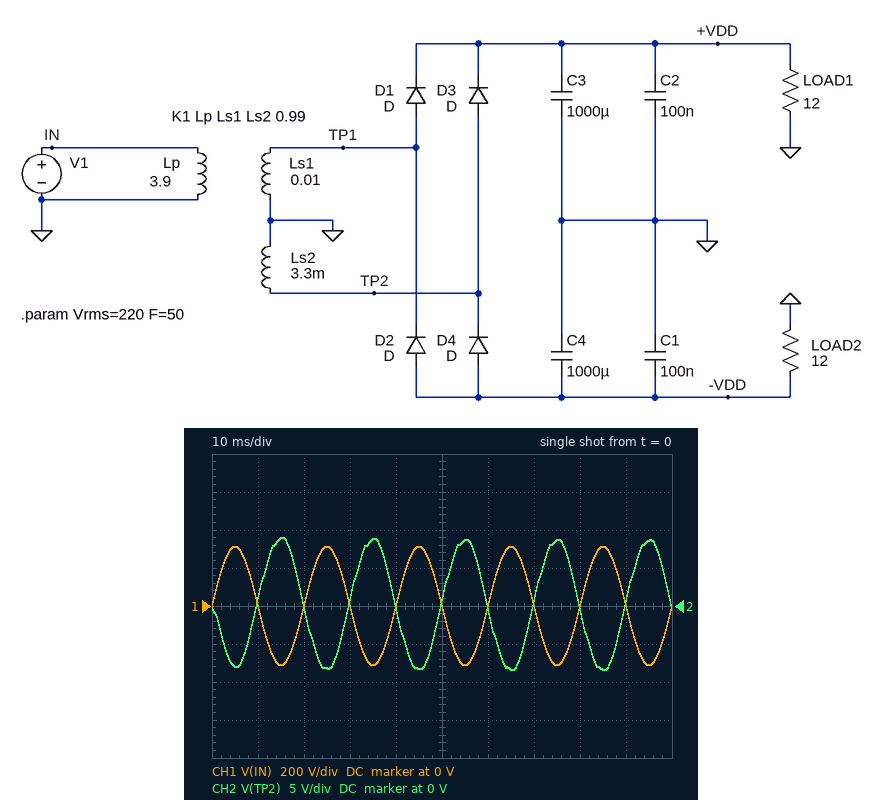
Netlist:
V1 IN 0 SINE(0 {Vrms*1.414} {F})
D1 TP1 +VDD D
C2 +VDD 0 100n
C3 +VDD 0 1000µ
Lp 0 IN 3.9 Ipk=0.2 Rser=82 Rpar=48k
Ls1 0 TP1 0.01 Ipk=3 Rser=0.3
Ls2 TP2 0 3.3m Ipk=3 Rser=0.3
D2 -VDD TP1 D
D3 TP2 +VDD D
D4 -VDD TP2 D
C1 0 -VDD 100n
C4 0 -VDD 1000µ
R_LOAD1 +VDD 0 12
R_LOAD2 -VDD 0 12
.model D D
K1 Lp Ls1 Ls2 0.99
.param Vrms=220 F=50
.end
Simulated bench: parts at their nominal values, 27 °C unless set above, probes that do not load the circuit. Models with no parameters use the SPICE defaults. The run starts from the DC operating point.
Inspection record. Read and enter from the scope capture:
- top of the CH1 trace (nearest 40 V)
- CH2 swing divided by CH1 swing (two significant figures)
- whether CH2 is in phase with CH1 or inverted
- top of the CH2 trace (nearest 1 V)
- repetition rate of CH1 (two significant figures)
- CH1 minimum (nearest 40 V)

320 V
0.028
inverted
9 V
50 Hz
-320 V
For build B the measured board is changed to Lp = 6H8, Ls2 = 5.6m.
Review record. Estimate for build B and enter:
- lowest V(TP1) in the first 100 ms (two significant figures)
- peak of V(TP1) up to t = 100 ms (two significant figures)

-12 V
11 V
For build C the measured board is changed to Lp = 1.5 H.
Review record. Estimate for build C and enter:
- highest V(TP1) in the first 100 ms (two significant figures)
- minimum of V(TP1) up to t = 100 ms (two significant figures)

23 V
-24 V
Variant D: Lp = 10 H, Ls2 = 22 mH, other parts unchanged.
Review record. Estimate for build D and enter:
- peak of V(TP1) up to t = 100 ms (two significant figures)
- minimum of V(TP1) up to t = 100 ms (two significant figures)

9.5 V
-9.8 V
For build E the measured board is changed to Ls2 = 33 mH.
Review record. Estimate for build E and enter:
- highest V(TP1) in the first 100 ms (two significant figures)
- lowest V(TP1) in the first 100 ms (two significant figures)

14 V
-15 V
